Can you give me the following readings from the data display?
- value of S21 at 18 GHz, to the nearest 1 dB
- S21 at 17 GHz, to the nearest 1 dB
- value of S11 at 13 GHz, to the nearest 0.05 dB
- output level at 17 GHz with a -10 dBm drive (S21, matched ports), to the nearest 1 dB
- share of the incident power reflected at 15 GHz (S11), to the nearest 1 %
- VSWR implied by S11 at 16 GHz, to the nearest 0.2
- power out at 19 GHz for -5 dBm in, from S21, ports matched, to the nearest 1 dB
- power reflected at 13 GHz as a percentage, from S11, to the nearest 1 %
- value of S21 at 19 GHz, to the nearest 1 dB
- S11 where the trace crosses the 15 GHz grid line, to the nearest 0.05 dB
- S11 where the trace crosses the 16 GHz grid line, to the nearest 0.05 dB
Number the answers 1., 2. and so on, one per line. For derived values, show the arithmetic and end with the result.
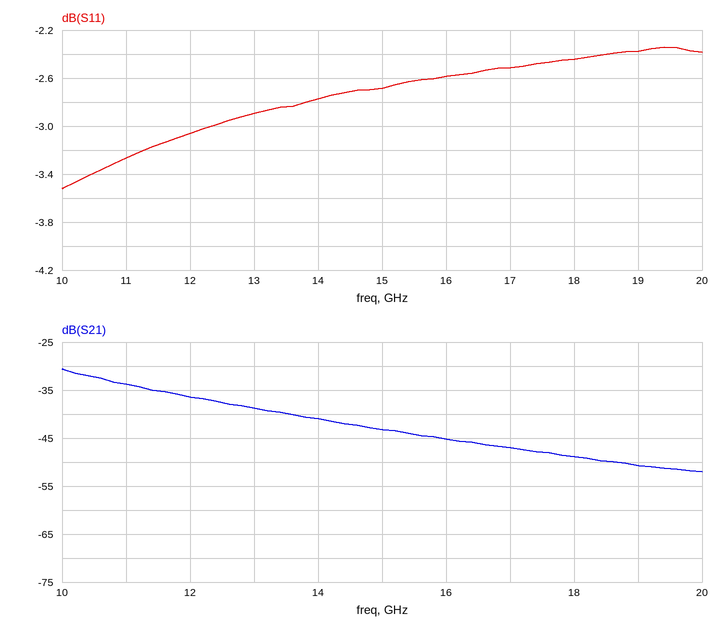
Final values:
1. -49 dB
2. -47 dB
3. -2.90 dB
4. -10 dBm + (-47 dB) = -57 dBm
5. 10^(-2.7/10) ≈ 54 %
6. |Γ| = 10^(-2.6/20) = 0.7413; VSWR = (1 + 0.7413)/(1 − 0.7413) ≈ 6.73, so 6.8 to the nearest 0.2
7. -5 dBm + (-51 dB) = -56 dBm
8. 10^(-2.9/10) ≈ 51 %
9. -51 dB
10. -2.70 dB
11. -2.60 dB
